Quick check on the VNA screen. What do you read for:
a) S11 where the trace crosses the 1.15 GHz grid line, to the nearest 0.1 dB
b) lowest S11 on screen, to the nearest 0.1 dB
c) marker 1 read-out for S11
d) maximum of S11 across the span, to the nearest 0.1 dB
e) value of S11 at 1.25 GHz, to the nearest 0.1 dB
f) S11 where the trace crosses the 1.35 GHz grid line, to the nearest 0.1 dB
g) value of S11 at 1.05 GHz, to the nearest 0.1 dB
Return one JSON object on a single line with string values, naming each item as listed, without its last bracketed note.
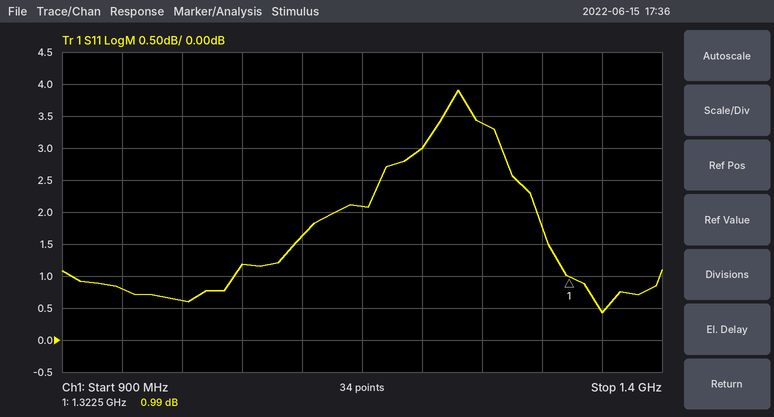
{"S11 where the trace crosses the 1.15 GHz grid line, to the nearest 0.1 dB": "2.1 dB", "lowest S11 on screen, to the nearest 0.1 dB": "0.4 dB", "marker 1 read-out for S11": "0.99 dB", "maximum of S11 across the span, to the nearest 0.1 dB": "3.9 dB", "value of S11 at 1.25 GHz, to the nearest 0.1 dB": "3.4 dB", "S11 where the trace crosses the 1.35 GHz grid line, to the nearest 0.1 dB": "0.4 dB", "value of S11 at 1.05 GHz, to the nearest 0.1 dB": "1.2 dB"}
